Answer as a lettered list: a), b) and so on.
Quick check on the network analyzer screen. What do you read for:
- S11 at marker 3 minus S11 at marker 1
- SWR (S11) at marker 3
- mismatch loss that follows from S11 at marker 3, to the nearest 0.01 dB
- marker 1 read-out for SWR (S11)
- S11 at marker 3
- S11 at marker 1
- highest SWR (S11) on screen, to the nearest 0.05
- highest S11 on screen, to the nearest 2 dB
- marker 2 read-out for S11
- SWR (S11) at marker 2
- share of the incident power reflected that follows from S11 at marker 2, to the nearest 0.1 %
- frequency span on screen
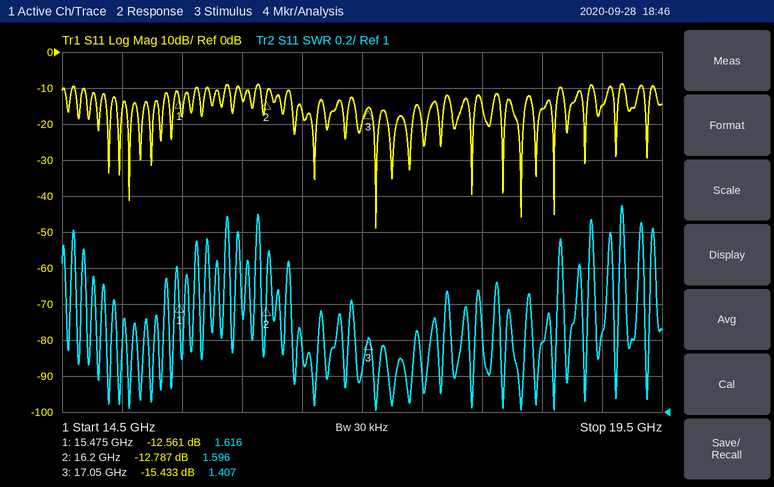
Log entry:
a) -2.872 dB
b) 1.407
c) 0.13 dB
d) 1.616
e) -15.433 dB
f) -12.561 dB
g) 2.15
h) -8 dB
i) -12.787 dB
j) 1.596
k) 5.3 %
l) 5 GHz
